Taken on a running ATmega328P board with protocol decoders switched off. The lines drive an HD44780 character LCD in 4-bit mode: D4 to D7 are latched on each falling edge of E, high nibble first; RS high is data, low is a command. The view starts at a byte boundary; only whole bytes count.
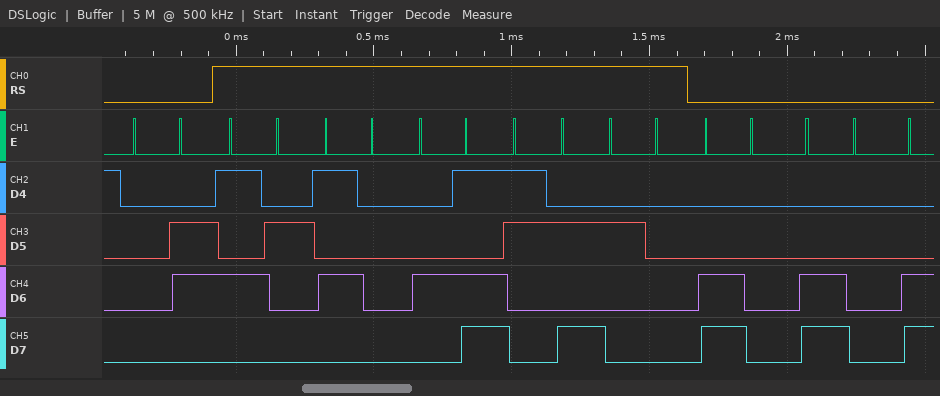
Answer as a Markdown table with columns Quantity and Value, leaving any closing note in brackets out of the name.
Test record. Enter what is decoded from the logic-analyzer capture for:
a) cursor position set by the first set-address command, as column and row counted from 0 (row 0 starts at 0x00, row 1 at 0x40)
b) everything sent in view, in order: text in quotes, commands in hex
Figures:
| Quantity | Value |
|---|---|
| cursor position set by the first set-address command, as column and row counted from 0 | column 0, row 1 |
| everything sent in view, in order: text in quotes, commands in hex | 0x06 "RPM: " 0xC0 0xC0 |
